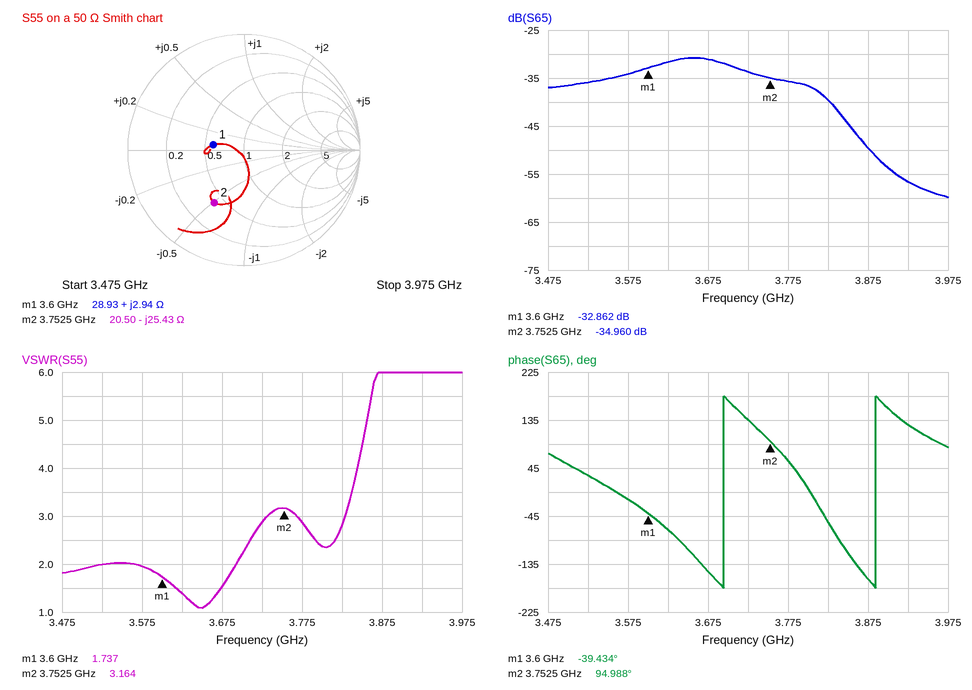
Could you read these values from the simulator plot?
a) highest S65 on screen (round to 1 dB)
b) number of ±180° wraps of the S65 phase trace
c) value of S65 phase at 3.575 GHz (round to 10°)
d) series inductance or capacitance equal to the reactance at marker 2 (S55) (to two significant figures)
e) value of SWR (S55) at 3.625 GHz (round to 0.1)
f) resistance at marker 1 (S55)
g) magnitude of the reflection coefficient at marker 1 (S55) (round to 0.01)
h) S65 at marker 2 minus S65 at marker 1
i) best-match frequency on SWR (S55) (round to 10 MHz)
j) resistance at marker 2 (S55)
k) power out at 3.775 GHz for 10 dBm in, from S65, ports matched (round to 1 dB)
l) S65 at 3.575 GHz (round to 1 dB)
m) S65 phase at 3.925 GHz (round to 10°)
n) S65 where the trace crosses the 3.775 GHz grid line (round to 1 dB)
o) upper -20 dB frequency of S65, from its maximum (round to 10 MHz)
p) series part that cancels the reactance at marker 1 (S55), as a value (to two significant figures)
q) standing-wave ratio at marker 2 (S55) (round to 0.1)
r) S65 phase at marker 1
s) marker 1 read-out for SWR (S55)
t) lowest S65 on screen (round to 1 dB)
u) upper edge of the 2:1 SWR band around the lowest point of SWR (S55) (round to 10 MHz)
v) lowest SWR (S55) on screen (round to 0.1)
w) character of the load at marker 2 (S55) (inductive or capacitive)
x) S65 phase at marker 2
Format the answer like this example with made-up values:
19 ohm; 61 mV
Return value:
-31 dB; 2; -10°; 1.7 pF; 1.4; 28.93 Ω; 0.27; -2.098 dB; 3.65 GHz; 20.50 Ω; -26 dBm; -34 dB; 130°; -36 dB; 3.88 GHz; 15 pF; 3.2; -39.434°; 1.737; -60 dB; 3.69 GHz; 1.1; capacitive; 94.988°
